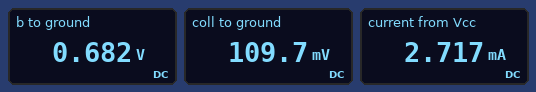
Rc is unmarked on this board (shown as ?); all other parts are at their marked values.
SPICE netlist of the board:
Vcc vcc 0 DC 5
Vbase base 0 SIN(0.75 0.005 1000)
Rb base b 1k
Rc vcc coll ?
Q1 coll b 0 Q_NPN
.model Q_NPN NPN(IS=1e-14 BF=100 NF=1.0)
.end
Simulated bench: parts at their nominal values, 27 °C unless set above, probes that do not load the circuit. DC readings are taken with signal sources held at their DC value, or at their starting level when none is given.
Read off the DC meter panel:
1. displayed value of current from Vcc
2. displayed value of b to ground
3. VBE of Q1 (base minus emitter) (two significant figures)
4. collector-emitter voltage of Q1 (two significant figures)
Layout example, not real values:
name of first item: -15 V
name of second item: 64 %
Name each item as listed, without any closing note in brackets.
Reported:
displayed value of current from Vcc: 2.717 mA
displayed value of b to ground: 0.682 V
VBE of Q1 (base minus emitter): 680 mV
collector-emitter voltage of Q1: 110 mV
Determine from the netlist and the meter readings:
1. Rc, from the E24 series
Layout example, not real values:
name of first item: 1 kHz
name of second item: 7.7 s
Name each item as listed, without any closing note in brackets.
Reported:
Rc, from the E24 series: 1.8 kΩ
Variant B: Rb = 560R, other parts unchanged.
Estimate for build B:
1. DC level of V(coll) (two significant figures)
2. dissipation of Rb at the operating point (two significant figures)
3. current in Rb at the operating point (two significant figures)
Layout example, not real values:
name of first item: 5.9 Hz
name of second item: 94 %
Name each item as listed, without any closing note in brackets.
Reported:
DC level of V(coll): 90 mV
dissipation of Rb at the operating point: 8.1 µW
current in Rb at the operating point: 120 µA
